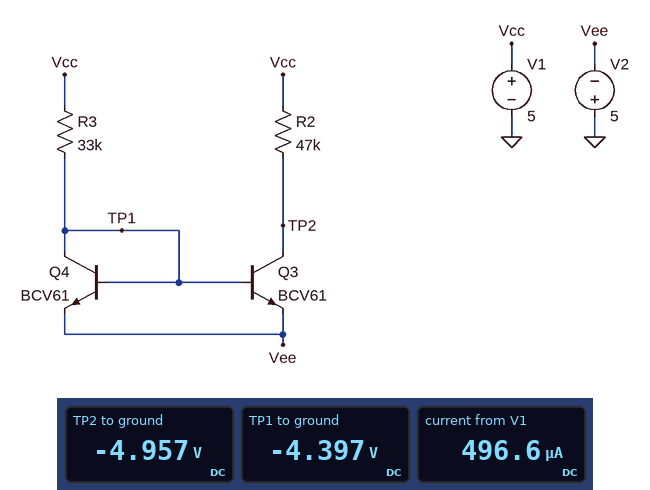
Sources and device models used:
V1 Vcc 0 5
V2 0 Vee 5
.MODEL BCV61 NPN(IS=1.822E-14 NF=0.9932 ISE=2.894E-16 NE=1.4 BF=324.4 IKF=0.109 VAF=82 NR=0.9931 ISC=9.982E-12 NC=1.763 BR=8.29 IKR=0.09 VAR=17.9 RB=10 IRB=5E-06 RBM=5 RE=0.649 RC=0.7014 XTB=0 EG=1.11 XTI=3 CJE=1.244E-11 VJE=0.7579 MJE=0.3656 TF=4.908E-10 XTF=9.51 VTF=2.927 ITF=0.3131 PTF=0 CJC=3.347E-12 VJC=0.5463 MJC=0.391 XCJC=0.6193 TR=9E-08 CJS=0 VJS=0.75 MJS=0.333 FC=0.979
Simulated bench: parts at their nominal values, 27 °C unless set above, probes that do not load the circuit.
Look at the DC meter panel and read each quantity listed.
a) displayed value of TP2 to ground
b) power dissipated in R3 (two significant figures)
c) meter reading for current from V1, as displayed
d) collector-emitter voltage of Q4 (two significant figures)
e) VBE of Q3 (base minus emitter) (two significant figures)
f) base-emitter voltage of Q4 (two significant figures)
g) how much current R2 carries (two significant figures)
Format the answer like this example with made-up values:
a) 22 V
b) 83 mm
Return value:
a) -4.957 V
b) 2.7 mW
c) 496.6 µA
d) 600 mV
e) 600 mV
f) 600 mV
g) 210 µA
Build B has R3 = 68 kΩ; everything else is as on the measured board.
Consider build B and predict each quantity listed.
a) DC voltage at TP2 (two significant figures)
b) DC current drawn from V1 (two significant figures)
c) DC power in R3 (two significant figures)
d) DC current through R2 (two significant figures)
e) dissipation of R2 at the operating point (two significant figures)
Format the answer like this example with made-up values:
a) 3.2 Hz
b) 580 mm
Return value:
a) -1.7 V
b) 280 µA
c) 1.3 mW
d) 140 µA
e) 950 µW
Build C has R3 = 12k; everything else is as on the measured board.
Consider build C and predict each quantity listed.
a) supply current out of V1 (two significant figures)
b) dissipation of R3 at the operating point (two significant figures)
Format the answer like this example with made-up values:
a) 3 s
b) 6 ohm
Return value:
a) 990 µA
b) 7.3 mW
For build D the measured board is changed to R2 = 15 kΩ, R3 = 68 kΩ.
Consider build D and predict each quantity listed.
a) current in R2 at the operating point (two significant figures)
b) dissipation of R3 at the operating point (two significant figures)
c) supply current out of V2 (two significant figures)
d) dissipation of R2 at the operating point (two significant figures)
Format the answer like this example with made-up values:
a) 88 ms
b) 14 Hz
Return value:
a) 150 µA
b) 1.3 mW
c) 290 µA
d) 340 µW
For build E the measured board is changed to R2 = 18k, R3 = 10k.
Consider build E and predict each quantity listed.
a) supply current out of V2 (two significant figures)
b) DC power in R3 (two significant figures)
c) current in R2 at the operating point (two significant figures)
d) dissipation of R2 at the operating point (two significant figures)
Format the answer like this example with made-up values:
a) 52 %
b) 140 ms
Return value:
a) 1.5 mA
b) 8.8 mW
c) 550 µA
d) 5.5 mW
